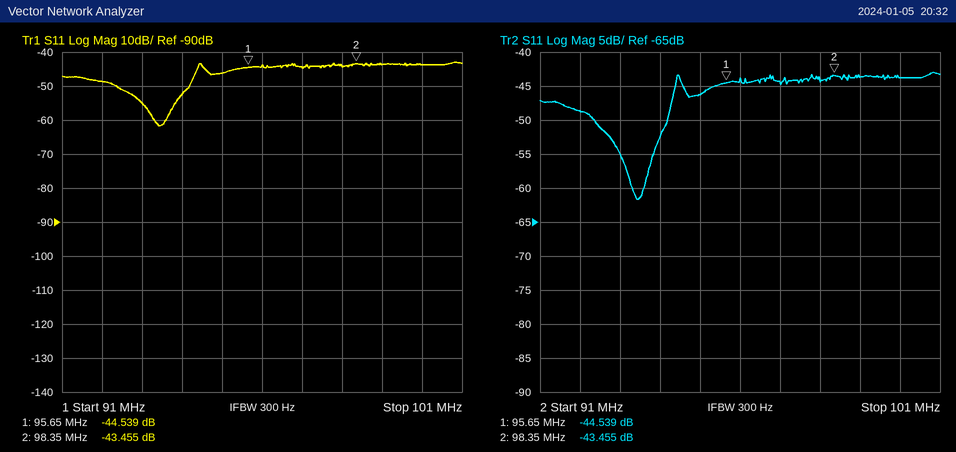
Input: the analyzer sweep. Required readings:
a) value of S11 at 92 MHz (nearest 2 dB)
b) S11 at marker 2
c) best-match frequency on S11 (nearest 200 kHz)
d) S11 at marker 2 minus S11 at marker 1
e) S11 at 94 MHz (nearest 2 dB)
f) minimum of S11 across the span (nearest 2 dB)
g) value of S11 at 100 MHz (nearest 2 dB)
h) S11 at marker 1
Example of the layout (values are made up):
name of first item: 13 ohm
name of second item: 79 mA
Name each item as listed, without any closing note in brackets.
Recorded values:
value of S11 at 92 MHz: -48 dB
S11 at marker 2: -43.455 dB
best-match frequency on S11: 93.4 MHz
S11 at marker 2 minus S11 at marker 1: 1.084 dB
S11 at 94 MHz: -52 dB
minimum of S11 across the span: -62 dB
value of S11 at 100 MHz: -44 dB
S11 at marker 1: -44.539 dB
